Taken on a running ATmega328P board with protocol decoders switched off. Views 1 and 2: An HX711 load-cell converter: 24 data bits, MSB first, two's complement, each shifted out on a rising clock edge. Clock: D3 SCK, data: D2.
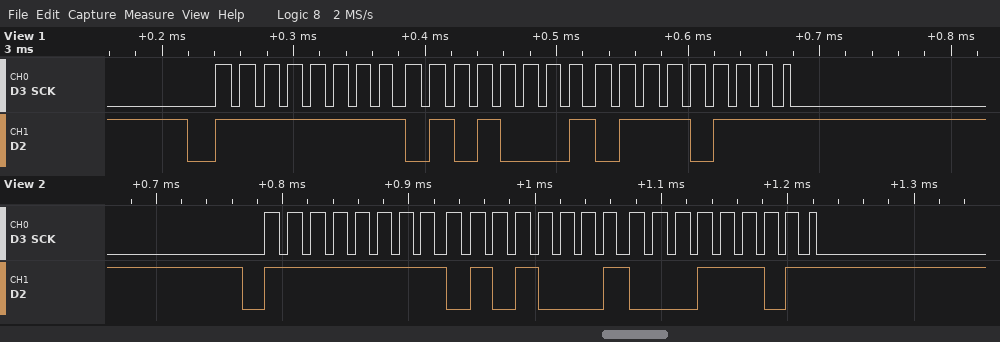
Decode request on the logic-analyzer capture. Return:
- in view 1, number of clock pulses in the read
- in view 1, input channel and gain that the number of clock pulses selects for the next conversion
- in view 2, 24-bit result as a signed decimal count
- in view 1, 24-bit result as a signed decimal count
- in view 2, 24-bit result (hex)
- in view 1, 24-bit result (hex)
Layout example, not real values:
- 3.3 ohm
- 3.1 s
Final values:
- 25
- channel A, gain 128
- -44771
- -44681
- 0xFF511D
- 0xFF5177
